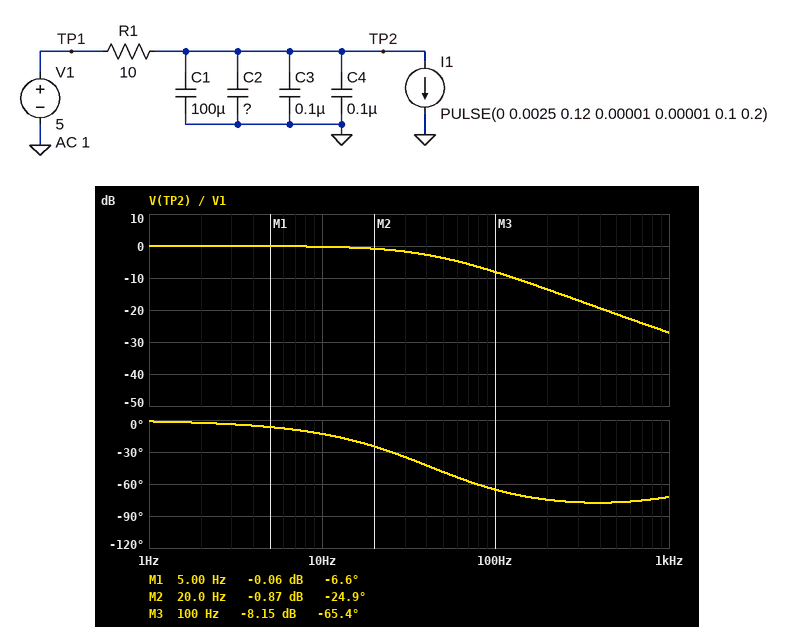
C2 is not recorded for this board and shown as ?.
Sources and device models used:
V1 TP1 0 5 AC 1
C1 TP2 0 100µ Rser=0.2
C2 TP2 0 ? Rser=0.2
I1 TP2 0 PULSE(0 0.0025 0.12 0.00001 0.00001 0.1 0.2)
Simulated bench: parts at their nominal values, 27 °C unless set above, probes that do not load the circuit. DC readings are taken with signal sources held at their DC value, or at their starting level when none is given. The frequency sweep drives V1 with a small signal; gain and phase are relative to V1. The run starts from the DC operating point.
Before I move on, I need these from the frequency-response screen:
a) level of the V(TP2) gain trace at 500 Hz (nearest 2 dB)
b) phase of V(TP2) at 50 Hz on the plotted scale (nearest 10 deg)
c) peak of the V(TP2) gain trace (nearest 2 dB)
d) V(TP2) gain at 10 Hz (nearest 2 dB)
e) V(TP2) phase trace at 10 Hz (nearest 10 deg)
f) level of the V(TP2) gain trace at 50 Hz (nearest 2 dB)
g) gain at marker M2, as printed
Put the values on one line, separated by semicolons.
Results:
-22 dB; -50 deg; 0 dB; 0 dB; -10 deg; -4 dB; -0.87 dB
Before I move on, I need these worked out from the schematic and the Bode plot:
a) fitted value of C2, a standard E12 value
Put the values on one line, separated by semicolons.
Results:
270 µF
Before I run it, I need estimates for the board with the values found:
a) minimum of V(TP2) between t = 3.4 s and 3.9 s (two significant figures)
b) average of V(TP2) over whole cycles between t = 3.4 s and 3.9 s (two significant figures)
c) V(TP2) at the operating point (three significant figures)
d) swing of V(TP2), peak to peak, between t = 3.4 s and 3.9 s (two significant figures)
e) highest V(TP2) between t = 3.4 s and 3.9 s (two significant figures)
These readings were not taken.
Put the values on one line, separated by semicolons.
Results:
5.0 V; 5.0 V; 5.00 V; 25 mV; 5.0 V
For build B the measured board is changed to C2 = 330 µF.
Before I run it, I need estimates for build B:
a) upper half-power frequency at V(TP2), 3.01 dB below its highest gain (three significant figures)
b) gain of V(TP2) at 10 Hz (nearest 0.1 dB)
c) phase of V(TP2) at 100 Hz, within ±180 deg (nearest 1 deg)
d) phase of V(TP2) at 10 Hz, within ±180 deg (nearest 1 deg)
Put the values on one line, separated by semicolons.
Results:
36.5 Hz; -0.3 dB; -68 deg; -15 deg
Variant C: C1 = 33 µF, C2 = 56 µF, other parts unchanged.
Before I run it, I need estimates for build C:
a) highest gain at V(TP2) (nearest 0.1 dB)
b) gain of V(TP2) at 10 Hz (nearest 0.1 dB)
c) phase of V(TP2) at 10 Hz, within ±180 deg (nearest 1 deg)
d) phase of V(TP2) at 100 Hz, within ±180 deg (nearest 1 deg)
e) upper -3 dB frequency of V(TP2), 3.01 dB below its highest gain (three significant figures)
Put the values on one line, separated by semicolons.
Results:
0 dB; 0 dB; -3 deg; -29 deg; 177 Hz
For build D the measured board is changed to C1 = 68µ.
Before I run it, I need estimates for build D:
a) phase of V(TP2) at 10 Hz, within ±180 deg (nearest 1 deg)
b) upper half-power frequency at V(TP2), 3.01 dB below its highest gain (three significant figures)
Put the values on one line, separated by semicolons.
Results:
-12 deg; 46.4 Hz
